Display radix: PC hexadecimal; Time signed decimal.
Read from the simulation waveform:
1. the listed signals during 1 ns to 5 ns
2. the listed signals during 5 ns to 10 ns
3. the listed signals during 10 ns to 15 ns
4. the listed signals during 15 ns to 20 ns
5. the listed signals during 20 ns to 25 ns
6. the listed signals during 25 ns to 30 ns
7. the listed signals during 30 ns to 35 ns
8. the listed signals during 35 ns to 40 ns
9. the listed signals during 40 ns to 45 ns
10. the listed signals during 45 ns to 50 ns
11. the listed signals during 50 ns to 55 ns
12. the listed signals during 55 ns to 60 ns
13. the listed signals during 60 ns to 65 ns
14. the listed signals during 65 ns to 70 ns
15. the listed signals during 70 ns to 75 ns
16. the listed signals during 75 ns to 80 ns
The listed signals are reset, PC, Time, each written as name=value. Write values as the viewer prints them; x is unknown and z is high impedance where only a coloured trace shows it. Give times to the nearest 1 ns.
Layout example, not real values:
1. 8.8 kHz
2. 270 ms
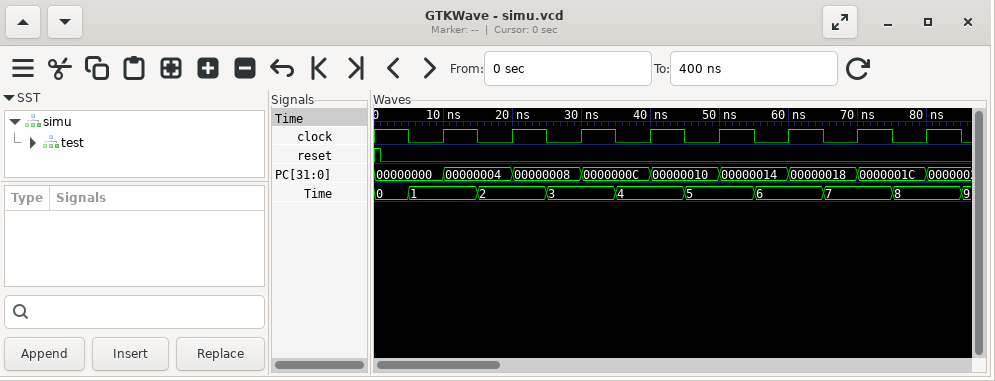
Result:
1. reset=0, PC=00000000, Time=0
2. reset=0, PC=00000000, Time=1
3. reset=0, PC=00000004, Time=1
4. reset=0, PC=00000004, Time=2
5. reset=0, PC=00000008, Time=2
6. reset=0, PC=00000008, Time=3
7. reset=0, PC=0000000C, Time=3
8. reset=0, PC=0000000C, Time=4
9. reset=0, PC=00000010, Time=4
10. reset=0, PC=00000010, Time=5
11. reset=0, PC=00000014, Time=5
12. reset=0, PC=00000014, Time=6
13. reset=0, PC=00000018, Time=6
14. reset=0, PC=00000018, Time=7
15. reset=0, PC=0000001C, Time=7
16. reset=0, PC=0000001C, Time=8
